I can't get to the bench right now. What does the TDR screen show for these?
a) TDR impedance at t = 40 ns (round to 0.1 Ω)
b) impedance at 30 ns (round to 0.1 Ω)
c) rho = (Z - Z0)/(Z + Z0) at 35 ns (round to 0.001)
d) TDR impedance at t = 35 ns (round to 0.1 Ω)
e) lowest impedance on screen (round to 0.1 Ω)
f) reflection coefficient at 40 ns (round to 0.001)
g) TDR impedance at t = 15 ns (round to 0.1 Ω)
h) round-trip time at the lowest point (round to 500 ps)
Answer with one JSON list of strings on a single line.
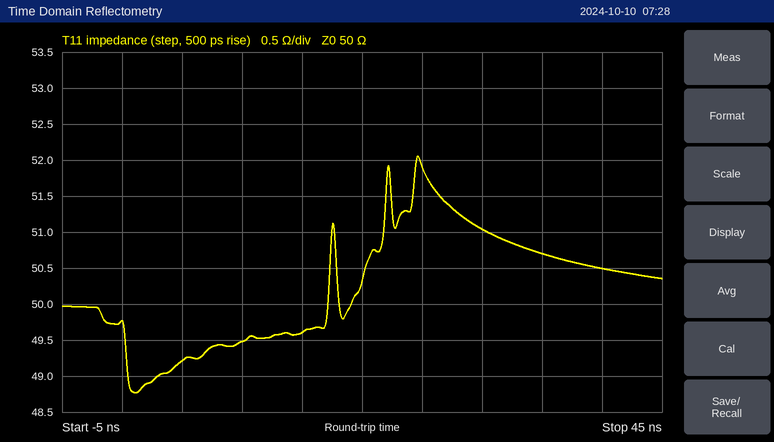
["50.5 Ω", "51.0 Ω", "+0.007", "50.7 Ω", "48.8 Ω", "+0.005", "49.6 Ω", "1.0 ns"]
